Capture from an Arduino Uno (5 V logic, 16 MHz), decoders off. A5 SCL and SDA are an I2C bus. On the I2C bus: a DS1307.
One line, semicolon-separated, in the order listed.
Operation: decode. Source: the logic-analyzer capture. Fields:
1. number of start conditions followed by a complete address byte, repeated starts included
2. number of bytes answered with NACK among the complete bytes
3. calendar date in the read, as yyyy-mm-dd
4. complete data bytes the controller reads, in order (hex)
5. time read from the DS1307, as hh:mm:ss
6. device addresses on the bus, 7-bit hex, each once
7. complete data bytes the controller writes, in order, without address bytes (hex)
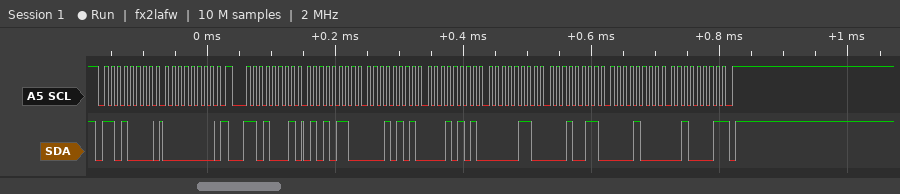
2; 1; 2021-08-13; 56 15 15 06 13 08 21; 15:15:56; 0x68; 00
